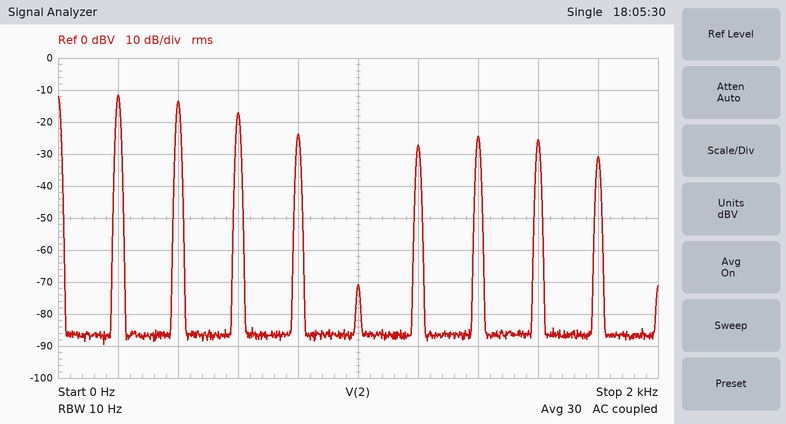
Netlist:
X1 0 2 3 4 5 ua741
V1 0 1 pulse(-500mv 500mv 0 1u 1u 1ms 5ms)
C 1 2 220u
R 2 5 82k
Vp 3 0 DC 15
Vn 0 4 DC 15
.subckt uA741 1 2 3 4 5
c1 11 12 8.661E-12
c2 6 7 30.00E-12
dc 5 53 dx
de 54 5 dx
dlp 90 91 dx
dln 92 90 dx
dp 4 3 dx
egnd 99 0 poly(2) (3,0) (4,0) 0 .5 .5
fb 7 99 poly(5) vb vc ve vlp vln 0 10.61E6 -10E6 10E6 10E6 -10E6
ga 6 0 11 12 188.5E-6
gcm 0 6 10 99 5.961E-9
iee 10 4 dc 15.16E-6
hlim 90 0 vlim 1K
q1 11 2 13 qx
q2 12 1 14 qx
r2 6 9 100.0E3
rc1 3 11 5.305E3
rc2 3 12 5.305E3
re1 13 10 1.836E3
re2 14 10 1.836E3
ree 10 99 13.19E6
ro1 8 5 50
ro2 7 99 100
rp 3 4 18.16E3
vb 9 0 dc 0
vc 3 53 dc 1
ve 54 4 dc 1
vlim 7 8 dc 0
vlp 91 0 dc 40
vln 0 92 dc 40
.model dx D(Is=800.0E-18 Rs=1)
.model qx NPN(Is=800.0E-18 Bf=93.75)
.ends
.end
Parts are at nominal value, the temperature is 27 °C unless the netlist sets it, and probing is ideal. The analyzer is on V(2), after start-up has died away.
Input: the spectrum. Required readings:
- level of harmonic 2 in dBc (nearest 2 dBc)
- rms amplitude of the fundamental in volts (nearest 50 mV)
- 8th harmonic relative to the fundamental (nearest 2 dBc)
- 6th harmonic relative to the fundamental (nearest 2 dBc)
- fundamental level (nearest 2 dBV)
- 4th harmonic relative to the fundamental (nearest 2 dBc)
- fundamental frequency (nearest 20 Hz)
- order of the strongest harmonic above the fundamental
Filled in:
-2 dBc
250 mV
-14 dBc
-16 dBc
-12 dBV
-12 dBc
200 Hz
2
